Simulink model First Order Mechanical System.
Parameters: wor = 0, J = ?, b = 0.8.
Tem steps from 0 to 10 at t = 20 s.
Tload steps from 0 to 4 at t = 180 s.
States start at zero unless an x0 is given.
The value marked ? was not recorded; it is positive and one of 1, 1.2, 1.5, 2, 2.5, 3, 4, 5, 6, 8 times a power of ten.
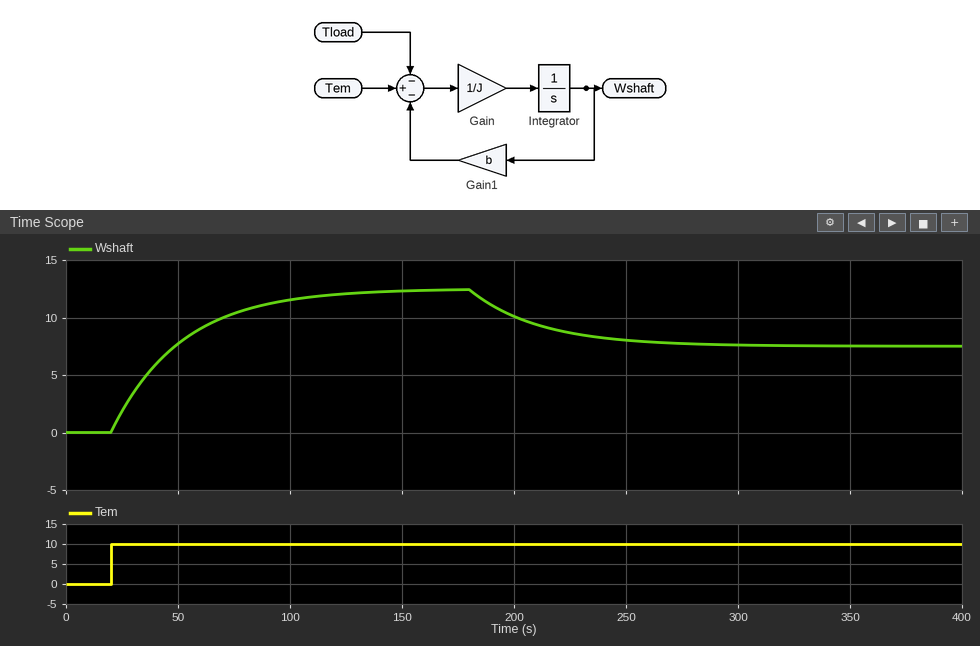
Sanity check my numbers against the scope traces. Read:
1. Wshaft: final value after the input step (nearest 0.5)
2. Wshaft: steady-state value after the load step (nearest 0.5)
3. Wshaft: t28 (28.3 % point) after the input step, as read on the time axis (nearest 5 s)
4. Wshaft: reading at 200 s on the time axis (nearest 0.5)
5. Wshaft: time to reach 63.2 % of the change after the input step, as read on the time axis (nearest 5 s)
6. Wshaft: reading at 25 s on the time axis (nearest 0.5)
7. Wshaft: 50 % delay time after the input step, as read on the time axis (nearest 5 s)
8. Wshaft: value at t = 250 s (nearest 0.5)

12.5
7.5
30 s
10.0
50 s
2.0
40 s
8.0
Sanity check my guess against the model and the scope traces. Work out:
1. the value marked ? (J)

25
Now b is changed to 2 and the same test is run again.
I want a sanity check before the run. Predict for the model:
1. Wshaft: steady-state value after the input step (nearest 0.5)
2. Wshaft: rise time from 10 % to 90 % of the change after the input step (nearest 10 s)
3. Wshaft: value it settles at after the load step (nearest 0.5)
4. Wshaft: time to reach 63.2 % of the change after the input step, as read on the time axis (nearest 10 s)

5.0
30 s
3.0
30 s
